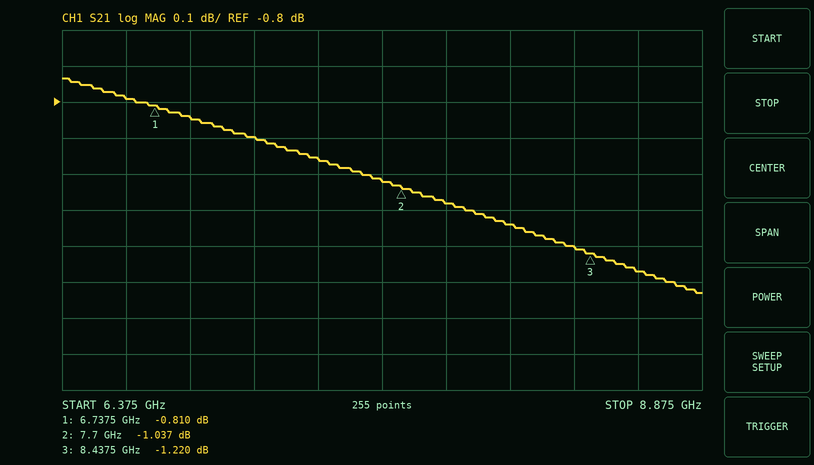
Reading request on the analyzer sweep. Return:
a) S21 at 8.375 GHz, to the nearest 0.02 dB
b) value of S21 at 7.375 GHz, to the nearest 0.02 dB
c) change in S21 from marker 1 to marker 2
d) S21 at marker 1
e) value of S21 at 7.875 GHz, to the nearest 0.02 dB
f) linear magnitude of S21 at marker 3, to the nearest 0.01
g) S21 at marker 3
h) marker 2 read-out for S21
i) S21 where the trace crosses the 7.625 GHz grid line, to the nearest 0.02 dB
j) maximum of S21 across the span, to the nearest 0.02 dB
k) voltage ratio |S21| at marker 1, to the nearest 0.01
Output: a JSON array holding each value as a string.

["-1.20 dB", "-0.96 dB", "-0.227 dB", "-0.810 dB", "-1.08 dB", "0.87", "-1.220 dB", "-1.037 dB", "-1.02 dB", "-0.74 dB", "0.91"]
